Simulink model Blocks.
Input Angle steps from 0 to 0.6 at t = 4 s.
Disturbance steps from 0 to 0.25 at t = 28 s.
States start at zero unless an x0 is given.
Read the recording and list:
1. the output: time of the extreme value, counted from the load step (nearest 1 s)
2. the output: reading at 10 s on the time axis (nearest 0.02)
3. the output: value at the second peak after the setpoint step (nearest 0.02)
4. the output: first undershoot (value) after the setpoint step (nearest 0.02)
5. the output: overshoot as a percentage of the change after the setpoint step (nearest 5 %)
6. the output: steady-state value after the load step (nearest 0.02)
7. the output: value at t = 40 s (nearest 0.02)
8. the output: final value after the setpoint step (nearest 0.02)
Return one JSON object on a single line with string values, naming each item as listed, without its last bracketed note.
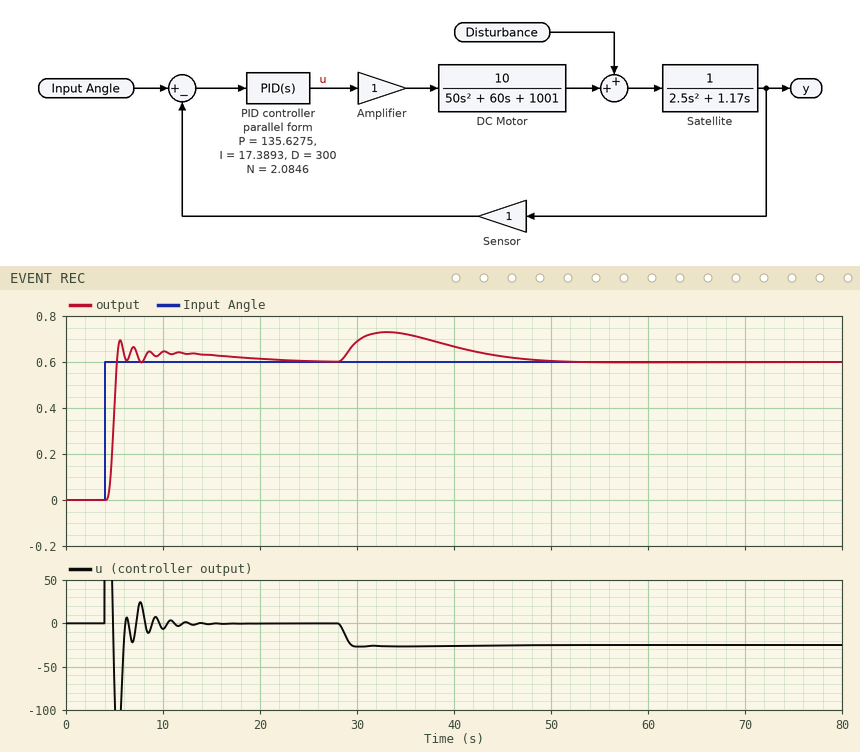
{"the output: time of the extreme value, counted from the load step": "5 s", "the output: reading at 10 s on the time axis": "0.64", "the output: value at the second peak after the setpoint step": "0.66", "the output: first undershoot (value) after the setpoint step": "0.60", "the output: overshoot as a percentage of the change after the setpoint step": "15 %", "the output: steady-state value after the load step": "0.60", "the output: value at t = 40 s": "0.66", "the output: final value after the setpoint step": "0.60"}
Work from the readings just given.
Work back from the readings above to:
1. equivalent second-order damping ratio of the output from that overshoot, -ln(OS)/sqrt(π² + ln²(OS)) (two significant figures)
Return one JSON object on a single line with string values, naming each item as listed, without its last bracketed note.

{"equivalent second-order damping ratio of the output from that overshoot, -ln(OS)/sqrt(π² + ln²(OS))": "0.52"}
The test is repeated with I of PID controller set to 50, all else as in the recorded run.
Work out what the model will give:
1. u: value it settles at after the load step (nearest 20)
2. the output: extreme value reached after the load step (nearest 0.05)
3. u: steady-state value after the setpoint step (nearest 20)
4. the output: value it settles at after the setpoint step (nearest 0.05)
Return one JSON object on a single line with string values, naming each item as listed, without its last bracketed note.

{"u: value it settles at after the load step": "-20", "the output: extreme value reached after the load step": "0.70", "u: steady-state value after the setpoint step": "0", "the output: value it settles at after the setpoint step": "0.60"}
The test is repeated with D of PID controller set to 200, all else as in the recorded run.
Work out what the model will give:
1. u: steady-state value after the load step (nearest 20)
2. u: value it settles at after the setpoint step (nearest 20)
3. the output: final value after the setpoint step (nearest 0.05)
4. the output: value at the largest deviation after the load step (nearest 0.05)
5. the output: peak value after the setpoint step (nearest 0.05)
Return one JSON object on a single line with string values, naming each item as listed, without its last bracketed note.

{"u: steady-state value after the load step": "-20", "u: value it settles at after the setpoint step": "0", "the output: final value after the setpoint step": "0.60", "the output: value at the largest deviation after the load step": "0.75", "the output: peak value after the setpoint step": "0.70"}
